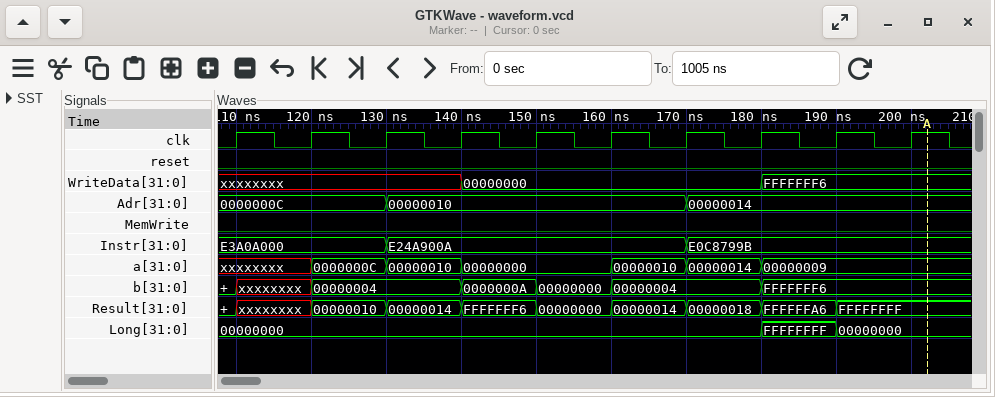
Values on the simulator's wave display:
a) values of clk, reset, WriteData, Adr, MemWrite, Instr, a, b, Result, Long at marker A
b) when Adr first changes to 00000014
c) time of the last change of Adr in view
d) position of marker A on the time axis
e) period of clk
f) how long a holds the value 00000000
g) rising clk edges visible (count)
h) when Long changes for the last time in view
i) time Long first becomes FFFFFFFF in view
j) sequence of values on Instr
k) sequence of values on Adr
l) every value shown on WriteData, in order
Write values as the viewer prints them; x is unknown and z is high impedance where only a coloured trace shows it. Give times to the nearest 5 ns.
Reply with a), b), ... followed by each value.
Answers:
a) clk=1, reset=0, WriteData=FFFFFFF6, Adr=00000014, MemWrite=0, Instr=E0C8799B, a=00000009, b=FFFFFFF6, Result=FFFFFFFF, Long=00000000
b) 170 ns
c) 170 ns
d) 200 ns
e) 10 ns
f) 20 ns
g) 10
h) 190 ns
i) 180 ns
j) E3A0A000, E24A900A, E0C8799B
k) 0000000C, 00000010, 00000014
l) xxxxxxxx, 00000000, FFFFFFF6
